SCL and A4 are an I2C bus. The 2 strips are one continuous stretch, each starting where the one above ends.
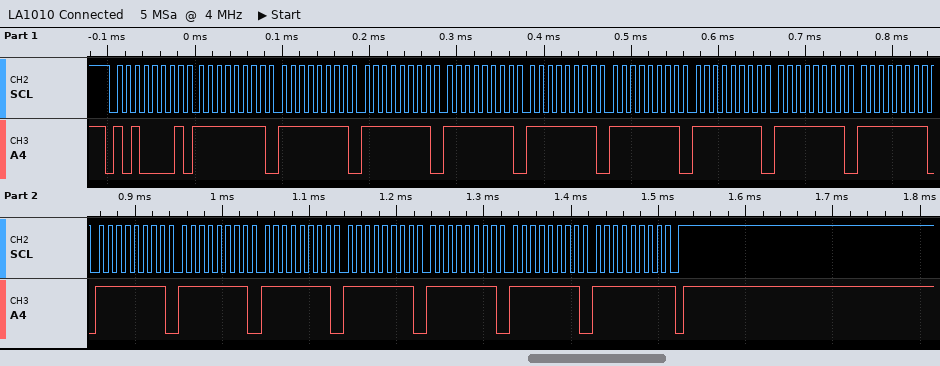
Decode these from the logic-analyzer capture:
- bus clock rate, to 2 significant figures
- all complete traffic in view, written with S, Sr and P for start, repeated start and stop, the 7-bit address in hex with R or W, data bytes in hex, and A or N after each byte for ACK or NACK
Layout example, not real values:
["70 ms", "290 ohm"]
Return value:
["100 kHz", "S 50R A FF A FF A FF A FF A FF A FF A FF A FF A FF A FF A FF A FF A FF A FF A FF A FF N P"]
